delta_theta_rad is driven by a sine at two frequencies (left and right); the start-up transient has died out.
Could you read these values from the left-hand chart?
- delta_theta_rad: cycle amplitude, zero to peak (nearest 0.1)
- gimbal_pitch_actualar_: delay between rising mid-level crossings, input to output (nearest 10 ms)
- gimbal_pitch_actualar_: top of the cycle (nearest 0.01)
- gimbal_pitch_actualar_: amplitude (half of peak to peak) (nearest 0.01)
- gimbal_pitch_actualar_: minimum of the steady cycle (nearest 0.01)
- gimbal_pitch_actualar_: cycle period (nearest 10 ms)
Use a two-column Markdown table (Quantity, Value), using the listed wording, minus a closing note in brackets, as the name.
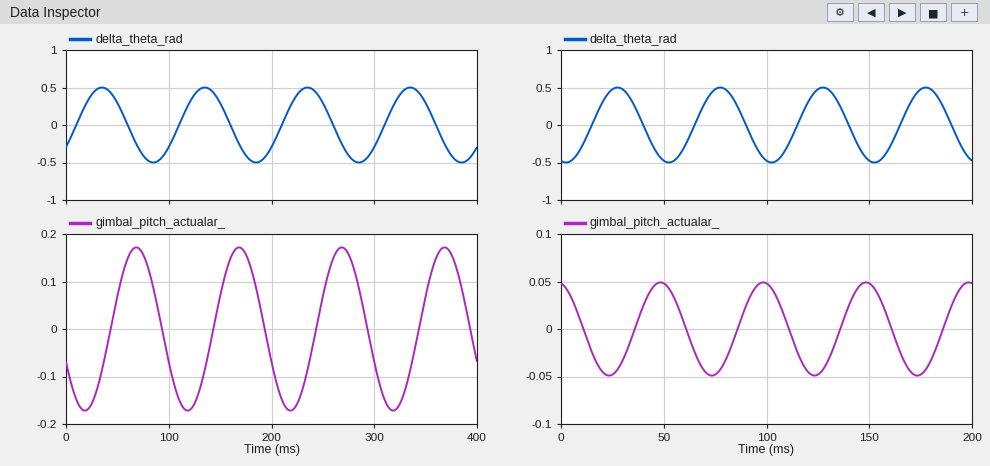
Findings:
| Quantity | Value |
|---|---|
| delta_theta_rad: cycle amplitude, zero to peak | 0.5 |
| gimbal_pitch_actualar_: delay between rising mid-level crossings, input to output | 30 ms |
| gimbal_pitch_actualar_: top of the cycle | 0.17 |
| gimbal_pitch_actualar_: amplitude (half of peak to peak) | 0.17 |
| gimbal_pitch_actualar_: minimum of the steady cycle | -0.17 |
| gimbal_pitch_actualar_: cycle period | 100 ms |
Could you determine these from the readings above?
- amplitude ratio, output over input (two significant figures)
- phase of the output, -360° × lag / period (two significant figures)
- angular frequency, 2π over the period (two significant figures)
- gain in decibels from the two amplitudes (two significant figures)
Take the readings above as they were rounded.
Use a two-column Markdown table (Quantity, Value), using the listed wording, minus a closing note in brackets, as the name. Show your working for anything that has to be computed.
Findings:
| Quantity | Value |
|---|---|
| amplitude ratio, output over input | 0.17 / 0.5 = 0.34 |
| phase of the output, -360° × lag / period | -360 × 30 / 100 = -110° |
| angular frequency, 2π over the period | 2π / 100 = 0.063 rad/ms |
| gain in decibels from the two amplitudes | 20 log10(0.17 / 0.5) = -9.4 dB |
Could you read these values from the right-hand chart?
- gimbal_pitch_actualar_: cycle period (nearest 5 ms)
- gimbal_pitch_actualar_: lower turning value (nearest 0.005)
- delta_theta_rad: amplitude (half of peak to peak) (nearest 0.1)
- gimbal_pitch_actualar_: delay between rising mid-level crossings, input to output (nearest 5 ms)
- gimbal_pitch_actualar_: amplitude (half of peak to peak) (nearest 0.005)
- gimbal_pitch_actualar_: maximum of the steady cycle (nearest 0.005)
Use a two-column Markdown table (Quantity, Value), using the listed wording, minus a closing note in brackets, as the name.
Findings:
| Quantity | Value |
|---|---|
| gimbal_pitch_actualar_: cycle period | 50 ms |
| gimbal_pitch_actualar_: lower turning value | -0.050 |
| delta_theta_rad: amplitude (half of peak to peak) | 0.5 |
| gimbal_pitch_actualar_: delay between rising mid-level crossings, input to output | 20 ms |
| gimbal_pitch_actualar_: amplitude (half of peak to peak) | 0.050 |
| gimbal_pitch_actualar_: maximum of the steady cycle | 0.050 |
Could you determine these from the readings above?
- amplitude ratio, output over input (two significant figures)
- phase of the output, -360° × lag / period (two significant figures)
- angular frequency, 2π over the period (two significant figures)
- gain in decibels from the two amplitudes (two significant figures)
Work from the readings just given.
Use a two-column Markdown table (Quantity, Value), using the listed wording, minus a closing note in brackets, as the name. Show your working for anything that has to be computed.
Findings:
| Quantity | Value |
|---|---|
| amplitude ratio, output over input | 0.05 / 0.5 = 0.10 |
| phase of the output, -360° × lag / period | -360 × 20 / 50 = -140° |
| angular frequency, 2π over the period | 2π / 50 = 0.13 rad/ms |
| gain in decibels from the two amplitudes | 20 log10(0.05 / 0.5) = -20 dB |
